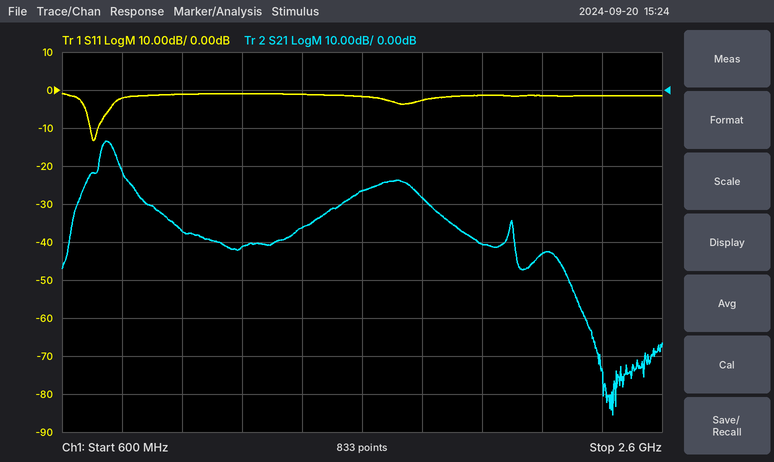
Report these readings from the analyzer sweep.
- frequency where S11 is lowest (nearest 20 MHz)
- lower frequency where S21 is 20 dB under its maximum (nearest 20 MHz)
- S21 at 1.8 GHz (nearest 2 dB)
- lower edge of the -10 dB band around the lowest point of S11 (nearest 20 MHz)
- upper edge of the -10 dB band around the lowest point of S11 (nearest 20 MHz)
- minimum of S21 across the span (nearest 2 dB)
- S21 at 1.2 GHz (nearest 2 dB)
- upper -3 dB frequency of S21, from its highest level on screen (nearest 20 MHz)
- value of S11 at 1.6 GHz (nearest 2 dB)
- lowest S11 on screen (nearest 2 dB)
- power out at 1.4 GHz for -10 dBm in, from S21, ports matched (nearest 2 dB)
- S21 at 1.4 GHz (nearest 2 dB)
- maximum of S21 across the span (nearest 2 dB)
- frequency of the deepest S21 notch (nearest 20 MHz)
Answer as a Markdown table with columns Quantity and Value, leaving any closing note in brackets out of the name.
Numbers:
| Quantity | Value |
|---|---|
| frequency where S11 is lowest | 700 MHz |
| lower frequency where S21 is 20 dB under its maximum | 640 MHz |
| S21 at 1.8 GHz | -28 dB |
| lower edge of the -10 dB band around the lowest point of S11 | 700 MHz |
| upper edge of the -10 dB band around the lowest point of S11 | 720 MHz |
| minimum of S21 across the span | -86 dB |
| S21 at 1.2 GHz | -42 dB |
| upper -3 dB frequency of S21, from its highest level on screen | 780 MHz |
| value of S11 at 1.6 GHz | -2 dB |
| lowest S11 on screen | -14 dB |
| power out at 1.4 GHz for -10 dBm in, from S21, ports matched | -46 dBm |
| S21 at 1.4 GHz | -36 dB |
| maximum of S21 across the span | -14 dB |
| frequency of the deepest S21 notch | 2.44 GHz |
